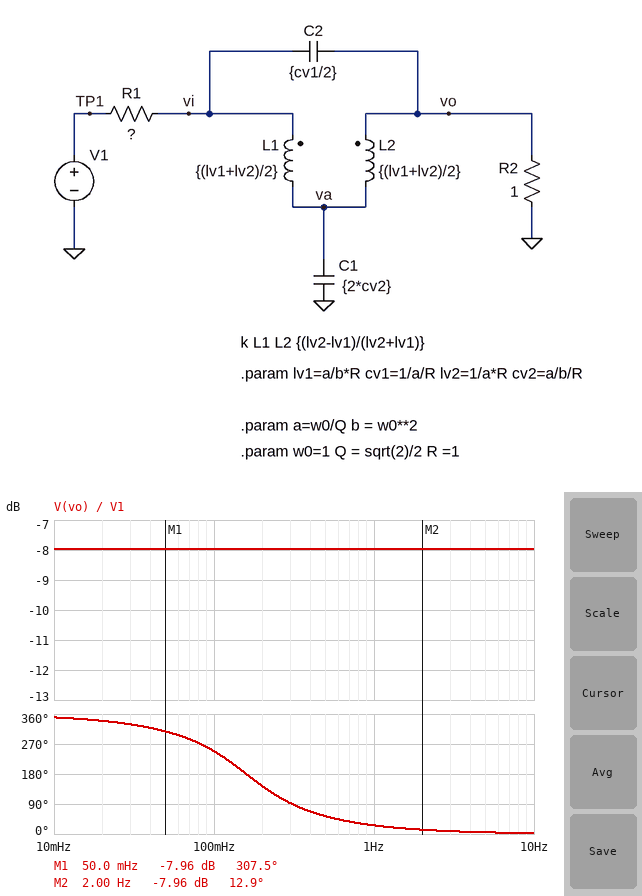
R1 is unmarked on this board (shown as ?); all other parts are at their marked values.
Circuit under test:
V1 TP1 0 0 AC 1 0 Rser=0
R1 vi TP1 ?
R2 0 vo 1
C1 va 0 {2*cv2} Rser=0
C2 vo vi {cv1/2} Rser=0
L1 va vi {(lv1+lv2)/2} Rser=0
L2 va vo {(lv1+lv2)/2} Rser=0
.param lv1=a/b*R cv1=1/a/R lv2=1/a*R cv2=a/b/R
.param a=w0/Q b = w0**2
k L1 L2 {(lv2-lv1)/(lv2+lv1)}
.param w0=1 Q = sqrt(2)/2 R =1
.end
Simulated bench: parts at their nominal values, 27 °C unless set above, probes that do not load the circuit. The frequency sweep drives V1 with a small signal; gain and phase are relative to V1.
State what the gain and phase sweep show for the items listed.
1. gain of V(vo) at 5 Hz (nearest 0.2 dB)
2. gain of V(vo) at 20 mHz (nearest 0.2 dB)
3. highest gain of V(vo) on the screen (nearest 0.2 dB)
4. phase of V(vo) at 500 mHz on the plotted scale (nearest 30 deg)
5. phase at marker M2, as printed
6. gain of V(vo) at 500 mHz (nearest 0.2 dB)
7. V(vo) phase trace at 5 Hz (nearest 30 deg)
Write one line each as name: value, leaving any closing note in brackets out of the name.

gain of V(vo) at 5 Hz: -8.0 dB
gain of V(vo) at 20 mHz: -8.0 dB
highest gain of V(vo) on the screen: -8.0 dB
phase of V(vo) at 500 mHz on the plotted scale: 60 deg
phase at marker M2, as printed: 12.9 deg
gain of V(vo) at 500 mHz: -8.0 dB
V(vo) phase trace at 5 Hz: 0 deg
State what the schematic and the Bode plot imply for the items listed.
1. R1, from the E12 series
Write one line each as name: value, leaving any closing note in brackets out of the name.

R1, from the E12 series: 1.5 Ω
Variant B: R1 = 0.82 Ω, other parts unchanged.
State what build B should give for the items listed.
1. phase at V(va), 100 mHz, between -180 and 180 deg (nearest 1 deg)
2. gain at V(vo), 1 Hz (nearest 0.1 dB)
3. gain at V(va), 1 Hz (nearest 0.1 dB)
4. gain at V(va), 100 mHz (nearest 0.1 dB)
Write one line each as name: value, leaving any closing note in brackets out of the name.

phase at V(va), 100 mHz, between -180 and 180 deg: -56 deg
gain at V(vo), 1 Hz: -5.2 dB
gain at V(va), 1 Hz: -37.1 dB
gain at V(va), 100 mHz: -5.8 dB
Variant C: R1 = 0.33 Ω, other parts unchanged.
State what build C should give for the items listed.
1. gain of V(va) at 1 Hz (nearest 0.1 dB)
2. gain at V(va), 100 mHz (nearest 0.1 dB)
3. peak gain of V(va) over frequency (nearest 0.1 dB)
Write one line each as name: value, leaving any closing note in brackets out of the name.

gain of V(va) at 1 Hz: -34.4 dB
gain at V(va), 100 mHz: -3.1 dB
peak gain of V(va) over frequency: -2.5 dB
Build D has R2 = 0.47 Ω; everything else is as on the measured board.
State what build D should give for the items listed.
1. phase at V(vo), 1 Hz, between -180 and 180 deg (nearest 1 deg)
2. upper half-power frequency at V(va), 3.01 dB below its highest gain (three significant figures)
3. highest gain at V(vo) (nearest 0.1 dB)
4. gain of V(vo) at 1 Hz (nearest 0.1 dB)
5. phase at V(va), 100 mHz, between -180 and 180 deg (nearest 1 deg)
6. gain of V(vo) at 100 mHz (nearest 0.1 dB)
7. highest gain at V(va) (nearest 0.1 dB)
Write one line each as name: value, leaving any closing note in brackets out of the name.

phase at V(vo), 1 Hz, between -180 and 180 deg: 23 deg
upper half-power frequency at V(va), 3.01 dB below its highest gain: 173 mHz
highest gain at V(vo): -11.2 dB
gain of V(vo) at 1 Hz: -12.2 dB
phase at V(va), 100 mHz, between -180 and 180 deg: -42 deg
gain of V(vo) at 100 mHz: -11.4 dB
highest gain at V(va): -6.7 dB
